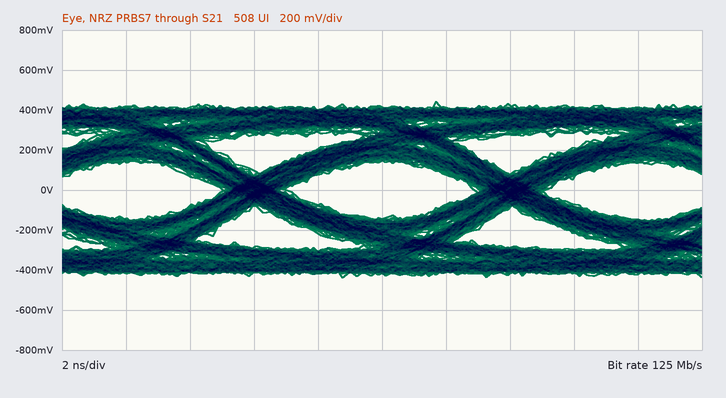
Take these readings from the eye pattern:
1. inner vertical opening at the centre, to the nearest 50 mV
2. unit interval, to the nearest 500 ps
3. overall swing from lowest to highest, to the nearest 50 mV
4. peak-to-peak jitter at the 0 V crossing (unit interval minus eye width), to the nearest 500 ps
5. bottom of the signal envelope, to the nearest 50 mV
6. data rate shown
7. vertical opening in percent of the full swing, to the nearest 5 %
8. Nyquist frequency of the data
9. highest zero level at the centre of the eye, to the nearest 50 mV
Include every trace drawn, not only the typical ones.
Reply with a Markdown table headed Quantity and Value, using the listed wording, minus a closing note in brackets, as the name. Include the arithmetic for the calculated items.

| Quantity | Value |
|---|---|
| inner vertical opening at the centre, to the nearest 50 mV | 300 mV |
| unit interval, to the nearest 500 ps | 8.0 ns |
| overall swing from lowest to highest, to the nearest 50 mV | 900 mV |
| peak-to-peak jitter at the 0 V crossing (unit interval minus eye width), to the nearest 500 ps | 2.0 ns |
| bottom of the signal envelope, to the nearest 50 mV | -450 mV |
| data rate shown | 125 Mb/s |
| vertical opening in percent of the full swing, to the nearest 5 % | 300 mV / 900 mV ≈ 33.3 %, so 35 % to the nearest 5 % |
| Nyquist frequency of the data | 62.5 MHz |
| highest zero level at the centre of the eye, to the nearest 50 mV | -150 mV |
